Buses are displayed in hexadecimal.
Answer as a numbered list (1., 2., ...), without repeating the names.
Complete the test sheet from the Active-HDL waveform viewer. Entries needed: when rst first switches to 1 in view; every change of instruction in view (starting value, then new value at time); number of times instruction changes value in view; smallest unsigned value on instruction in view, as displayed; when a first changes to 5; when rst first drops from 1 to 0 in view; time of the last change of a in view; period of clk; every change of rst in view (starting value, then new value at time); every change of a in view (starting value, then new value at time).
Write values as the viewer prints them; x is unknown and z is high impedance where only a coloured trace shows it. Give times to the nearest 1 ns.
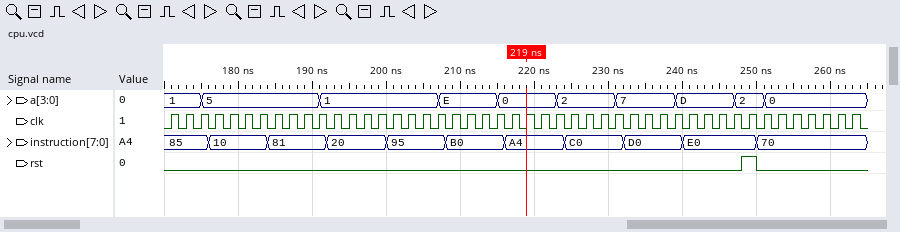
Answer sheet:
1. 248 ns
2. 85, 10 at 176 ns, 81 at 184 ns, 20 at 192 ns, 95 at 200 ns, B0 at 208 ns, A4 at 216 ns, C0 at 224 ns, D0 at 232 ns, E0 at 240 ns, 70 at 250 ns
3. 10
4. 10
5. 175 ns
6. 250 ns
7. 251 ns
8. 2 ns
9. 0, 1 at 248 ns, 0 at 250 ns
10. 1, 5 at 175 ns, 1 at 191 ns, E at 207 ns, 0 at 215 ns, 2 at 223 ns, 7 at 231 ns, D at 239 ns, 2 at 247 ns, 0 at 251 ns
